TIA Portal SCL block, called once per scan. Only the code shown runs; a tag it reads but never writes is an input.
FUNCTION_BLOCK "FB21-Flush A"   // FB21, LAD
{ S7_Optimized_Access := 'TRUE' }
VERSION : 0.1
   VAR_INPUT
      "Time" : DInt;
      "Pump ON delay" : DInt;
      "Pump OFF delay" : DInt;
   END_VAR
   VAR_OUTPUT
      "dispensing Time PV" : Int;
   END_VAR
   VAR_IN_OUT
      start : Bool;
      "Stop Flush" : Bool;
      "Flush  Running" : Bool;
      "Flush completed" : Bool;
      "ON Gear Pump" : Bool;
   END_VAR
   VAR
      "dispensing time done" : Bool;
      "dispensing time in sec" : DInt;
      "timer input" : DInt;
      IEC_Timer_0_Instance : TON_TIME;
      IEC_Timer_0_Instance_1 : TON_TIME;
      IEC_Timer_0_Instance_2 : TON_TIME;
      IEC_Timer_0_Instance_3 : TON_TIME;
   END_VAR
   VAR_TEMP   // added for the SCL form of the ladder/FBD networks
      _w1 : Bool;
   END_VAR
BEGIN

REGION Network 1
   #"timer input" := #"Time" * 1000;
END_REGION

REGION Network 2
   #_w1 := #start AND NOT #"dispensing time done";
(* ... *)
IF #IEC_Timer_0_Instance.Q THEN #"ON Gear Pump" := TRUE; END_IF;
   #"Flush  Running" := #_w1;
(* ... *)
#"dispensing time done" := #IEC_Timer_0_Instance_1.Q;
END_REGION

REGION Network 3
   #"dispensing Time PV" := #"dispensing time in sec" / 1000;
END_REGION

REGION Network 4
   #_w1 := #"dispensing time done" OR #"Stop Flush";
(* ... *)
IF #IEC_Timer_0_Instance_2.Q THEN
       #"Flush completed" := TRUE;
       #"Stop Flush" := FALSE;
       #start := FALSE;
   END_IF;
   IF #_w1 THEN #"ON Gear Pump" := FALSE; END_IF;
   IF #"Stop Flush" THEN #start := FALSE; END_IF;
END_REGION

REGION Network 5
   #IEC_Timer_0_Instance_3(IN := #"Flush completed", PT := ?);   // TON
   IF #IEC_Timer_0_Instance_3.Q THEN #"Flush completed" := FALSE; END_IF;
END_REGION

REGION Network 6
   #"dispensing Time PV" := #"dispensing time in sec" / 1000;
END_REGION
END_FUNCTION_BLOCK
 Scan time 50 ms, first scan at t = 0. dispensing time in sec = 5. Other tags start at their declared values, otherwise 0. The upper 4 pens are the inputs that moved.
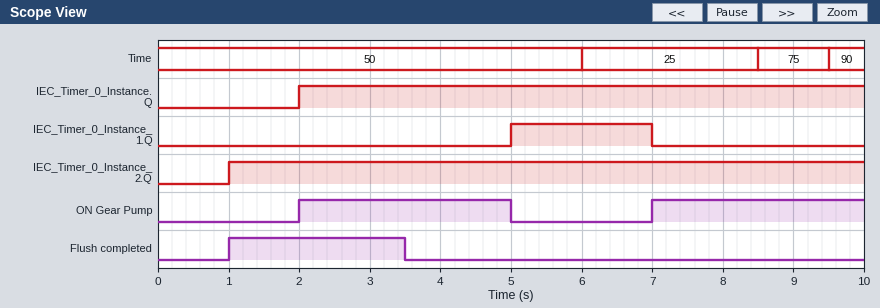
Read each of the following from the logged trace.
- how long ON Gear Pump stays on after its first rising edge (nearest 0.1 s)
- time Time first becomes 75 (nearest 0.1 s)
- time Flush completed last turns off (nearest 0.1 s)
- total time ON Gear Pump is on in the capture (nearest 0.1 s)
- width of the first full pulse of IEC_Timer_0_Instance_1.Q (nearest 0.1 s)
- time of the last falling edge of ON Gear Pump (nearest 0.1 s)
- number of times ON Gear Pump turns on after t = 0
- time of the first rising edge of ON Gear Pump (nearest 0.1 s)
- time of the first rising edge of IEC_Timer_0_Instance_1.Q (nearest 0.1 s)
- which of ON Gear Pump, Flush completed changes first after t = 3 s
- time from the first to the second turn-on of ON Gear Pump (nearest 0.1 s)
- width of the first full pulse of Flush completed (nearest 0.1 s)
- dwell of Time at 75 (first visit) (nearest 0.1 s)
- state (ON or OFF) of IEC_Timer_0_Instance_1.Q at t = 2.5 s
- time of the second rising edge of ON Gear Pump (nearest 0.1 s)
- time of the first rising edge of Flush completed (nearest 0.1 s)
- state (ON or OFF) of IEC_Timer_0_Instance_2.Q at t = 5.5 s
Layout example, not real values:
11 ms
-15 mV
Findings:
3.0 s
8.5 s
3.5 s
6.0 s
2.0 s
5.0 s
2
2.0 s
5.0 s
Flush completed
5.0 s
2.5 s
1.0 s
OFF
7.0 s
1.0 s
ON
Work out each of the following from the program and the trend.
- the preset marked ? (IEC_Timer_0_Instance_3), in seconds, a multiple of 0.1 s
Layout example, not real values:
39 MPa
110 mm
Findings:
2.5 s
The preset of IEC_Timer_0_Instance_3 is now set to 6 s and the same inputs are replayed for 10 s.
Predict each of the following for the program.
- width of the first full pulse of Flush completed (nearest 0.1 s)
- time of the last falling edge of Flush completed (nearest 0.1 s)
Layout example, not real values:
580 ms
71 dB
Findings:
6.0 s
7.0 s
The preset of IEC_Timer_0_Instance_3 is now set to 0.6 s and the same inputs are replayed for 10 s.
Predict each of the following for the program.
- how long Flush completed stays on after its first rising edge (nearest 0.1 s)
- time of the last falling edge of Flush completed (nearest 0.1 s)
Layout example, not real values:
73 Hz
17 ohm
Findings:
0.6 s
1.6 s
